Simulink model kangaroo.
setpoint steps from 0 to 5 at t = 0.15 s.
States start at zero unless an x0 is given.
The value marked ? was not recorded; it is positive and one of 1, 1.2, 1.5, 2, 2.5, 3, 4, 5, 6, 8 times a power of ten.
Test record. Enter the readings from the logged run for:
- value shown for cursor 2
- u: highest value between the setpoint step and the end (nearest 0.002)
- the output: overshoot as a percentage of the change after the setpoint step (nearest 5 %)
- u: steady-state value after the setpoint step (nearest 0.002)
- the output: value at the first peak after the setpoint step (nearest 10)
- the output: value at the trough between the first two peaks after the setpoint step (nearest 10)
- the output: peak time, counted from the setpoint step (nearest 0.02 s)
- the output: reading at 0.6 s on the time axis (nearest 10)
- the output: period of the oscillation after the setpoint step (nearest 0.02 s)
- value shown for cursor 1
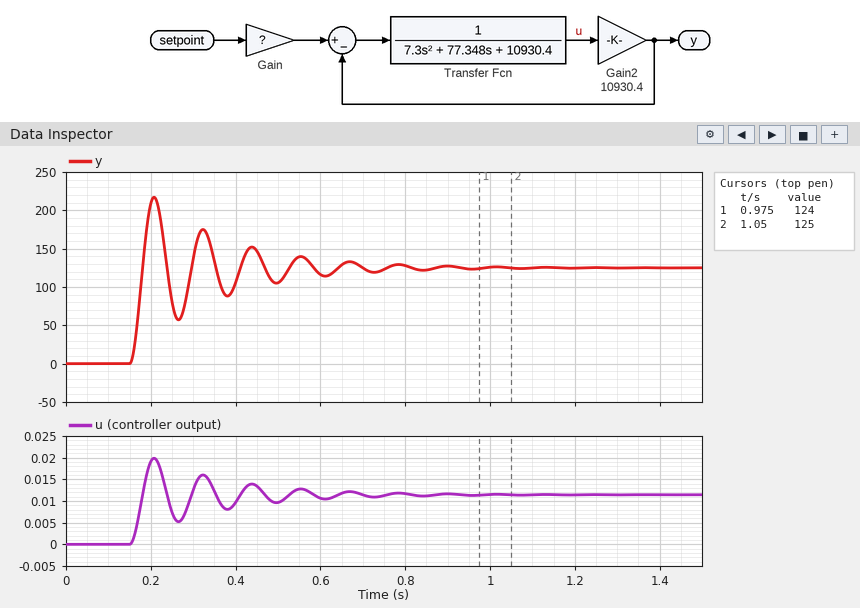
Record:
125
0.020
75 %
0.012
220
60
0.06 s
120
0.12 s
124
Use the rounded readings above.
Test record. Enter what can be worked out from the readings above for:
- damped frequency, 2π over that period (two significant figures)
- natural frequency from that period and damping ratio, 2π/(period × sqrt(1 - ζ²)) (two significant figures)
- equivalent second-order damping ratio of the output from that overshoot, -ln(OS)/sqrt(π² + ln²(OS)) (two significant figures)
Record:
52 rad/s
53 rad/s
0.091
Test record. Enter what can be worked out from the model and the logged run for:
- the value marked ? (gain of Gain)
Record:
50
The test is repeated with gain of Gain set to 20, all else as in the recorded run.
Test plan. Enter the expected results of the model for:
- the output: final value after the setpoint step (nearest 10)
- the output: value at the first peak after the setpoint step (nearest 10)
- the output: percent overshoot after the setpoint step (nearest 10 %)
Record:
50
90
70 %
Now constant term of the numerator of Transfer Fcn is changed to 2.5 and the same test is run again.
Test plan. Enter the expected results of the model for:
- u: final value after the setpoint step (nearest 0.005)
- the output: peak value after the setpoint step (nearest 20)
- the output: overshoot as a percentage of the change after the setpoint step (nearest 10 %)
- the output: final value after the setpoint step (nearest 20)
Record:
0.015
320
80 %
180
